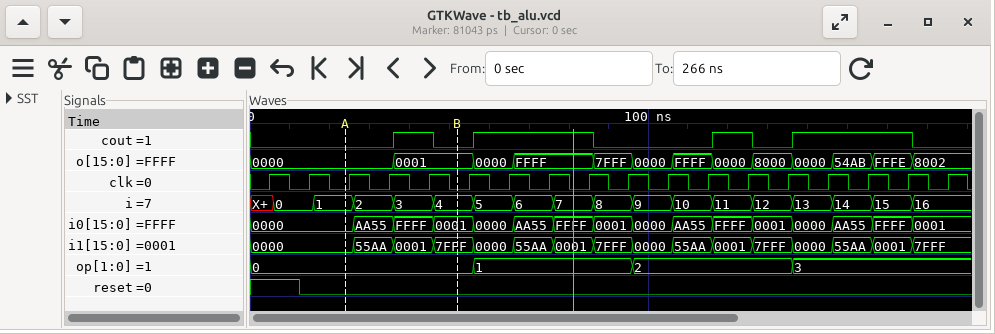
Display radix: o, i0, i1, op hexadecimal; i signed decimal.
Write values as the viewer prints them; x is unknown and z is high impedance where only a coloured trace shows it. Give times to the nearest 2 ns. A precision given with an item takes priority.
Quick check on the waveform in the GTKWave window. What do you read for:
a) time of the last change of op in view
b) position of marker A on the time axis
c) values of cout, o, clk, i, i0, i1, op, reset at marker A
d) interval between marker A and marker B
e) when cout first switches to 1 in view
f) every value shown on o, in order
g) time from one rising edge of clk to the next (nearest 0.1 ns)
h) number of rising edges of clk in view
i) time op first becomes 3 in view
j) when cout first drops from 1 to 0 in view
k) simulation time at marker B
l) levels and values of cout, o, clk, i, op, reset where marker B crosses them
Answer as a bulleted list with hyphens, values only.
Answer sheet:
- 136 ns
- 24 ns
- cout=0, o=0000, clk=0, i=1, i0=0000, i1=0000, op=0, reset=0
- 28 ns
- 36 ns
- 0000, 0001, 0000, FFFF, 7FFF, 0000, FFFF, 0000, 8000, 0000, 54AB, FFFE, 8002
- 10 ns
- 18
- 136 ns
- 46 ns
- 52 ns
- cout=0, o=0001, clk=0, i=4, op=0, reset=0
